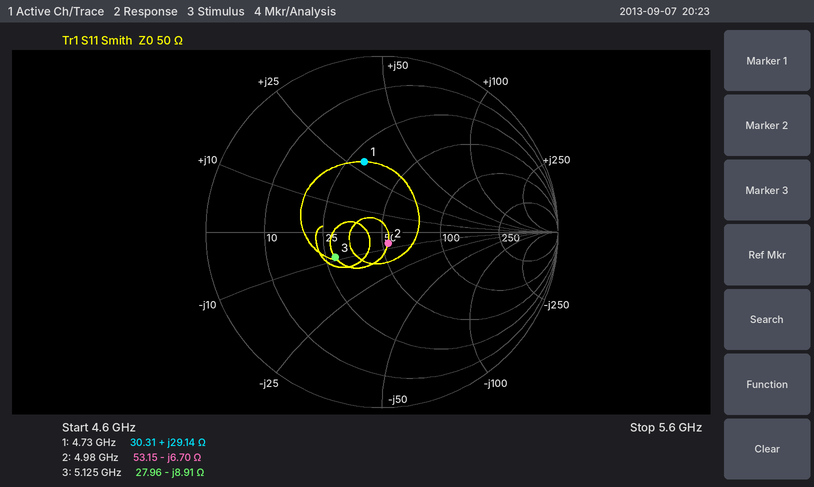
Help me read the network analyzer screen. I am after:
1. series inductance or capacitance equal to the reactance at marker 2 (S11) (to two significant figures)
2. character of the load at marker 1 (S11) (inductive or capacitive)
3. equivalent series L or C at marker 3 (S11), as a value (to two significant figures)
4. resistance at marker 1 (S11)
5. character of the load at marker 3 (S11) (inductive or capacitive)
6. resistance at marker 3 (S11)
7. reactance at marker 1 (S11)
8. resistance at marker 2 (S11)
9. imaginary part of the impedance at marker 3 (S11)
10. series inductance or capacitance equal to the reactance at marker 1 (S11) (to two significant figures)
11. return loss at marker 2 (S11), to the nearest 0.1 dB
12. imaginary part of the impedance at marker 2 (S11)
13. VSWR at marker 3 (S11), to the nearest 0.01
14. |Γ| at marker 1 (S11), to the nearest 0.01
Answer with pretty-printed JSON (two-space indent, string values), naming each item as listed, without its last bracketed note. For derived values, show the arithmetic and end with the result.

{
  "series inductance or capacitance equal to the reactance at marker 2 (S11)": "C = 1/(2π × 4.98 GHz × 6.7 Ω) ≈ 4.8 pF",
  "character of the load at marker 1 (S11)": "inductive",
  "equivalent series L or C at marker 3 (S11), as a value": "C = 1/(2π × 5.125 GHz × 8.91 Ω) ≈ 3.5 pF",
  "resistance at marker 1": "30.31 Ω",
  "character of the load at marker 3 (S11)": "capacitive",
  "resistance at marker 3": "27.96 Ω",
  "reactance at marker 1": "+29.14 Ω",
  "resistance at marker 2": "53.15 Ω",
  "imaginary part of the impedance at marker 3": "-8.91 Ω",
  "series inductance or capacitance equal to the reactance at marker 1 (S11)": "L = 29.14 Ω/(2π × 4.73 GHz) ≈ 981 pH, so 980 pH to two significant figures",
  "return loss at marker 2 (S11), to the nearest 0.1 dB": "22.9 dB",
  "imaginary part of the impedance at marker 2": "-6.70 Ω",
  "VSWR at marker 3 (S11), to the nearest 0.01": "1.87",
  "|Γ| at marker 1 (S11), to the nearest 0.01": "0.41"
}
